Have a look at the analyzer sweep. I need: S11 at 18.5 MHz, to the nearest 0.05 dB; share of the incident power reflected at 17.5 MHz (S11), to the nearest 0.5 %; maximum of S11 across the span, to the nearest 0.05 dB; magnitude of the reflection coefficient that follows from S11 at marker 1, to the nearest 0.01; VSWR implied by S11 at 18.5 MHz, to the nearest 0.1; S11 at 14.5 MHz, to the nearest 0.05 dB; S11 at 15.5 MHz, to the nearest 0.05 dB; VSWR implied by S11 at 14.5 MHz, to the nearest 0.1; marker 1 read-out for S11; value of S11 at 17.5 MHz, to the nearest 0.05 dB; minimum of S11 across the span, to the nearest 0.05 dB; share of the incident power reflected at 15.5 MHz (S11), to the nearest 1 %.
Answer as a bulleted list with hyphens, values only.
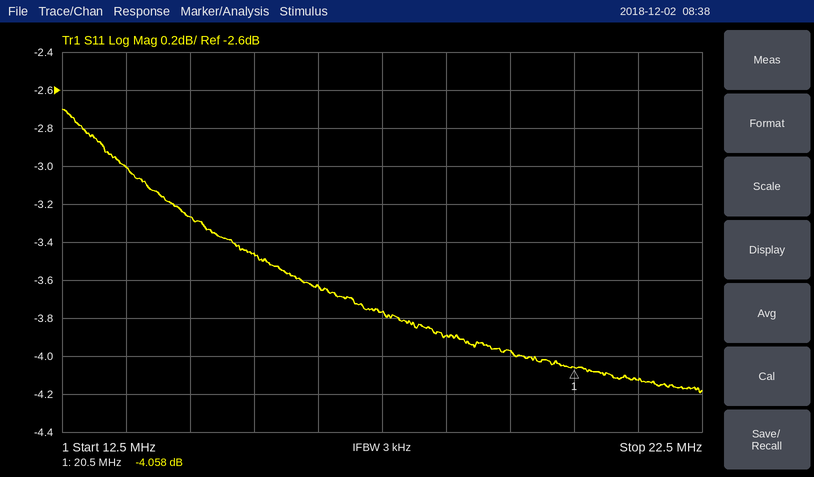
- -3.90 dB
- 42.0 %
- -2.70 dB
- 0.63
- 4.5
- -3.25 dB
- -3.45 dB
- 5.4
- -4.058 dB
- -3.75 dB
- -4.20 dB
- 45 %
